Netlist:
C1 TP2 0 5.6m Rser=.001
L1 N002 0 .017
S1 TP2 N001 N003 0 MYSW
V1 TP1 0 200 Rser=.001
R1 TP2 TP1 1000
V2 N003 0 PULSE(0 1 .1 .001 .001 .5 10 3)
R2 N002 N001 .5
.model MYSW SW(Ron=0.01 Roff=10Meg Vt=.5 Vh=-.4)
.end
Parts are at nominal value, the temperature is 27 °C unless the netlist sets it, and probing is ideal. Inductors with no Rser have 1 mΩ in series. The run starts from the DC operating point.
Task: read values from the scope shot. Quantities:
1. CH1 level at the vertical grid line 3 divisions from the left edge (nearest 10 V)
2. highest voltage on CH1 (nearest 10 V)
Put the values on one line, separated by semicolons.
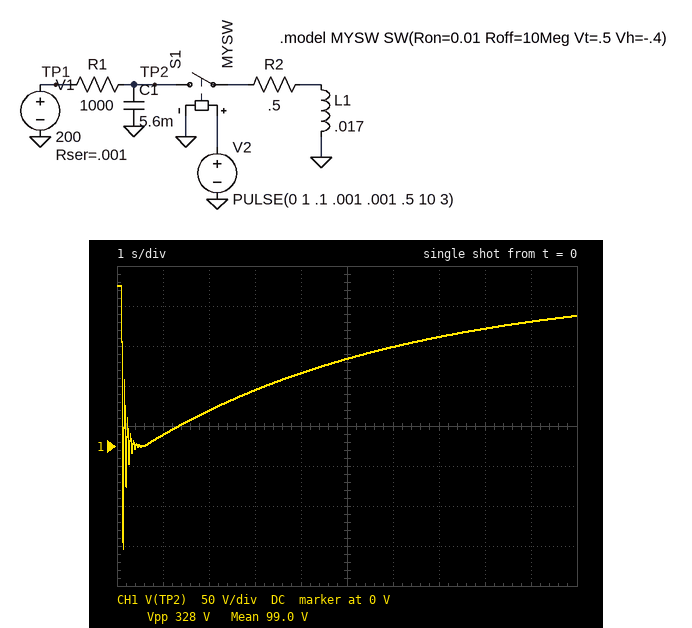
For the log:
70 V; 200 V
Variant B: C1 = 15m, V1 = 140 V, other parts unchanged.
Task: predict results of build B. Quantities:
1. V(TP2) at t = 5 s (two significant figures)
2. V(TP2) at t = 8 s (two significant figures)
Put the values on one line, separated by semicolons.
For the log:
36 V; 55 V
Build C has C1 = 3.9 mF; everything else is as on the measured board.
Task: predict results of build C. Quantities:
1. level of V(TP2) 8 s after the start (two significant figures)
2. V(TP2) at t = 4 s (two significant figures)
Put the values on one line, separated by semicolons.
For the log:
170 V; 120 V
